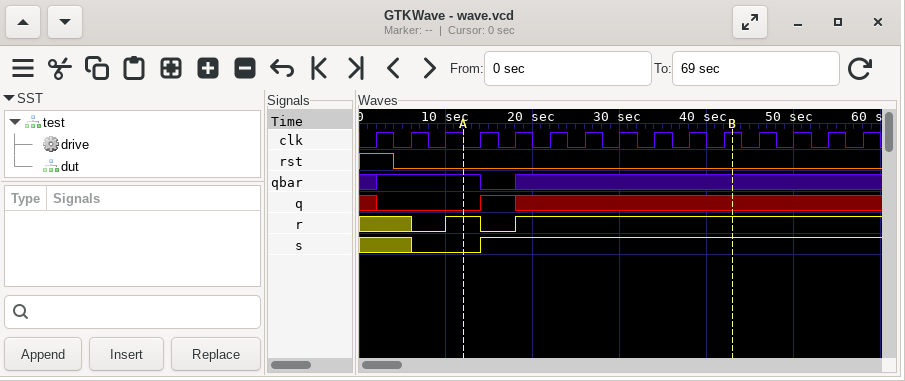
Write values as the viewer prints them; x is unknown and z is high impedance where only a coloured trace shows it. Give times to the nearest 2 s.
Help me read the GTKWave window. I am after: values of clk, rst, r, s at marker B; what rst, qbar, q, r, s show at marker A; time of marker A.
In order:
clk=1, rst=0, r=1, s=1
rst=0, qbar=1, q=0, r=1, s=0
12 s
